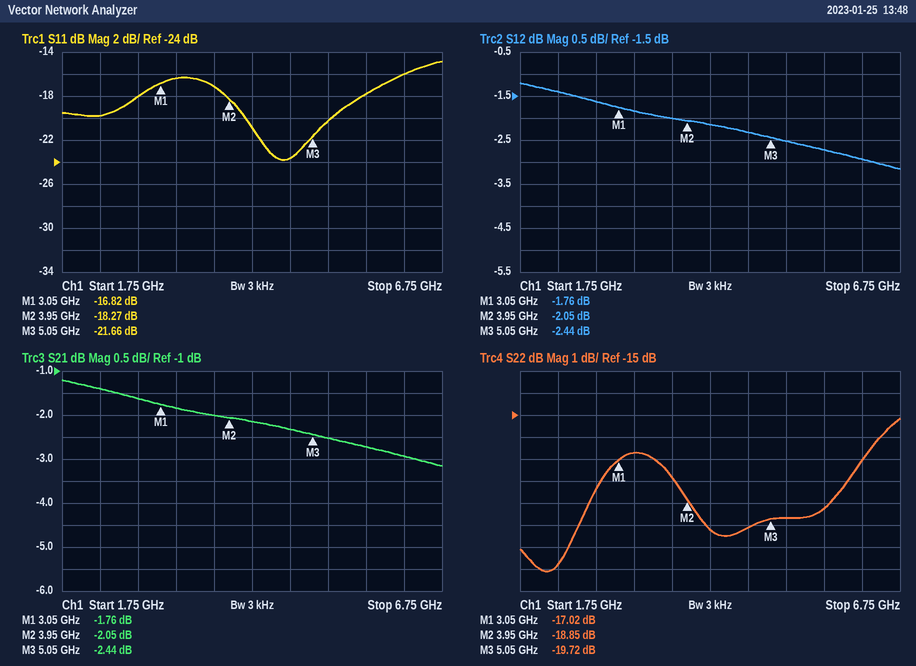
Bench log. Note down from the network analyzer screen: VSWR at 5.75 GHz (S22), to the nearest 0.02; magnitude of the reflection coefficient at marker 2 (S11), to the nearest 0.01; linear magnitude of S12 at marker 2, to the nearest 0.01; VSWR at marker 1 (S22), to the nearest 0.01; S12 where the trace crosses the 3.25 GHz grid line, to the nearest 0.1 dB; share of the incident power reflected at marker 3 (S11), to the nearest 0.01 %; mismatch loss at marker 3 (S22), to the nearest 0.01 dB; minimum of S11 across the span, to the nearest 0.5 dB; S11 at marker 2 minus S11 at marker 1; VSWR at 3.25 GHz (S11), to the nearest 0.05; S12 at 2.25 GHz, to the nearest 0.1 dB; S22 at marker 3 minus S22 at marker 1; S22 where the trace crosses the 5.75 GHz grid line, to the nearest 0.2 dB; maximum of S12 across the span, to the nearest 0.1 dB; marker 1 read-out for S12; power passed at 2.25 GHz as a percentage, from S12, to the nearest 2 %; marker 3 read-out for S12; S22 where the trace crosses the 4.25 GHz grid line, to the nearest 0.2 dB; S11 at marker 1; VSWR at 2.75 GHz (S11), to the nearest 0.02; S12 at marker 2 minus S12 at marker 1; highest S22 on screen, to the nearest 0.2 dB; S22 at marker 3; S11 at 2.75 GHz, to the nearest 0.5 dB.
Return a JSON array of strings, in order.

["1.24", "0.12", "0.79", "1.33", "-1.8 dB", "0.68 %", "0.05 dB", "-24.0 dB", "-1.45 dB", "1.35", "-1.4 dB", "-2.70 dB", "-19.2 dB", "-1.2 dB", "-1.76 dB", "72 %", "-2.44 dB", "-20.2 dB", "-16.82 dB", "1.28", "-0.29 dB", "-15.2 dB", "-19.72 dB", "-18.0 dB"]
